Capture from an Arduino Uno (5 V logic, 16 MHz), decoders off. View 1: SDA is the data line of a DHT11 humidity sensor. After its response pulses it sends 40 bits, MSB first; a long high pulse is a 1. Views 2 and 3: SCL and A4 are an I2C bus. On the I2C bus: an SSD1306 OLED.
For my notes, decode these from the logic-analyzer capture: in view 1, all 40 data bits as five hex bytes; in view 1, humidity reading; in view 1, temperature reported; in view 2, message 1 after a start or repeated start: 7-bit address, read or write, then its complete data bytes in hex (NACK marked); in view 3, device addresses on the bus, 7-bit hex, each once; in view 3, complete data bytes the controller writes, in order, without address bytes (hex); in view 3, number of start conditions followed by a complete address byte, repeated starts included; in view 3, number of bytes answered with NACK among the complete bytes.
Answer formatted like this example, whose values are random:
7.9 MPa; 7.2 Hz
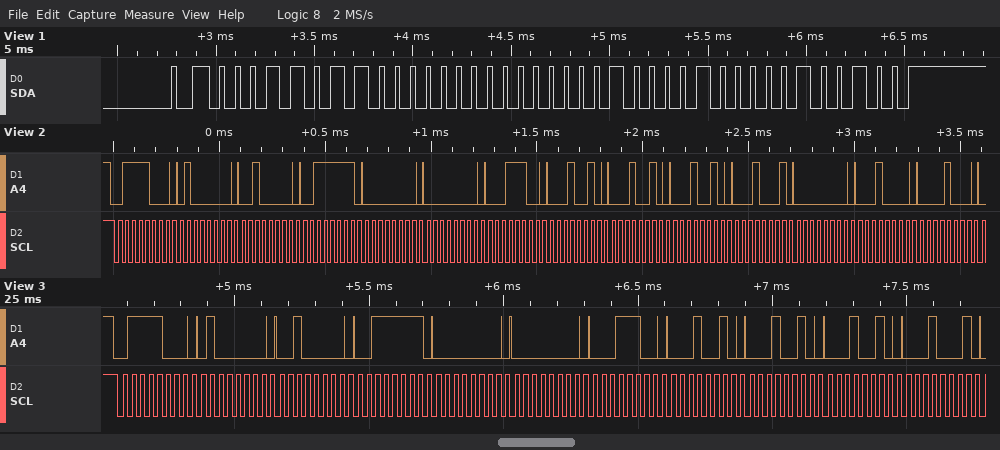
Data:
1B 00 01 08 24; 27 %; 1.8 °C; 0x3C write: 40 20 3F 00 00 1C 12 12 12 11 00 10 08; 0x3C; 40 20 3F 00 00 1C 12 12 12 11; 1; 0
